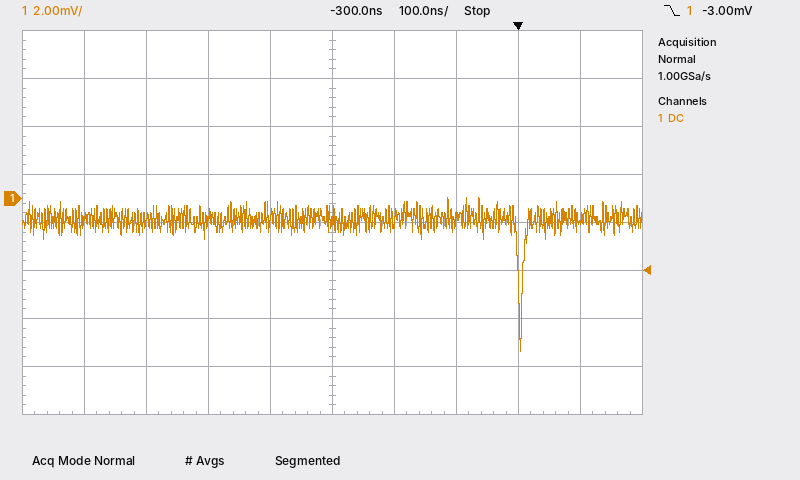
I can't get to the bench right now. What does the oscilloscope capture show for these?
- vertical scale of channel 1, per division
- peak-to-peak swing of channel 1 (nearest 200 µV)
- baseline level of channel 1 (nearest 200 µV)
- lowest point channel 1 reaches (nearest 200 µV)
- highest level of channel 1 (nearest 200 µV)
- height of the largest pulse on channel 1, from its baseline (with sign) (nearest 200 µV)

2 mV
6.4 mV
-800 µV
-6.4 mV
0.0 mV
-5.6 mV
